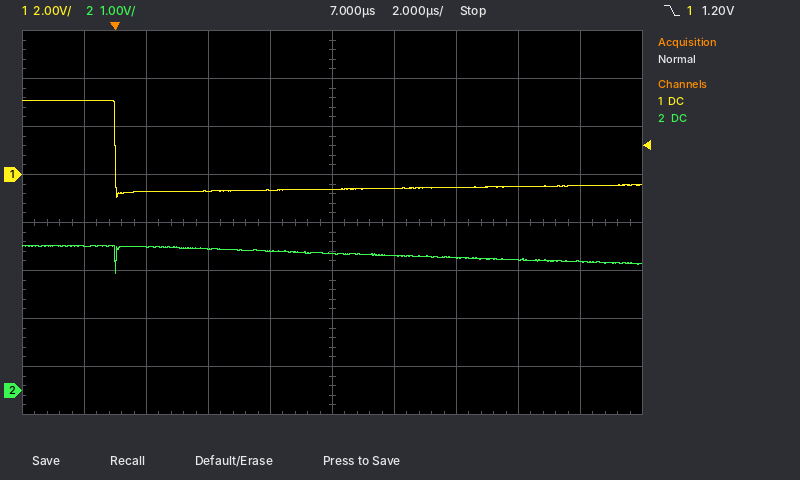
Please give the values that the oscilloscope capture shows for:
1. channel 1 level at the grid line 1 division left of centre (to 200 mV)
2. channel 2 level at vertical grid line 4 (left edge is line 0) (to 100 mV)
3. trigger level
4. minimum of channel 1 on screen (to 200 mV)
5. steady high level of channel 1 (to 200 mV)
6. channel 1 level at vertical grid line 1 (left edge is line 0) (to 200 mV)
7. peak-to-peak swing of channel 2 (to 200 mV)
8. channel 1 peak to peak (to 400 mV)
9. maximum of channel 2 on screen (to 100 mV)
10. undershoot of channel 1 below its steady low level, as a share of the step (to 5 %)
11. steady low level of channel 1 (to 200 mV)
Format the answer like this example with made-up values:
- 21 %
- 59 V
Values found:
- -600 mV
- 2.9 V
- 1.20 V
- -1.0 V
- 3.0 V
- 3.0 V
- 600 mV
- 4.0 V
- 3.0 V
- 10 %
- -600 mV
